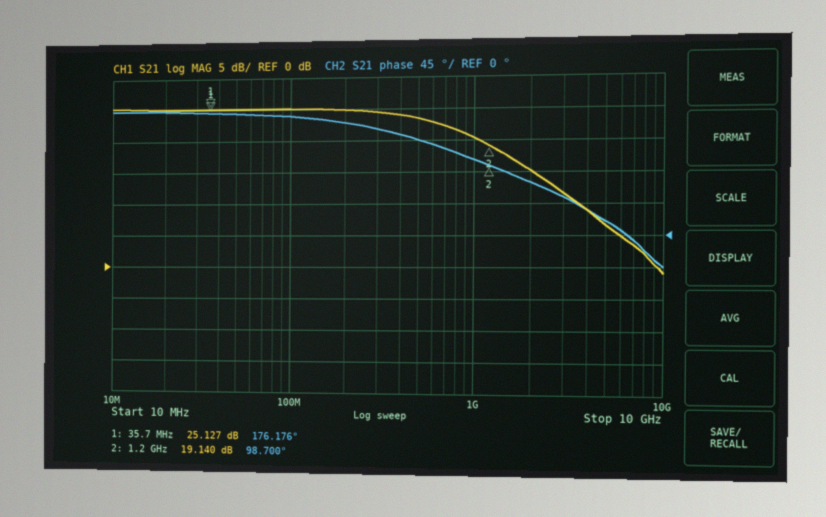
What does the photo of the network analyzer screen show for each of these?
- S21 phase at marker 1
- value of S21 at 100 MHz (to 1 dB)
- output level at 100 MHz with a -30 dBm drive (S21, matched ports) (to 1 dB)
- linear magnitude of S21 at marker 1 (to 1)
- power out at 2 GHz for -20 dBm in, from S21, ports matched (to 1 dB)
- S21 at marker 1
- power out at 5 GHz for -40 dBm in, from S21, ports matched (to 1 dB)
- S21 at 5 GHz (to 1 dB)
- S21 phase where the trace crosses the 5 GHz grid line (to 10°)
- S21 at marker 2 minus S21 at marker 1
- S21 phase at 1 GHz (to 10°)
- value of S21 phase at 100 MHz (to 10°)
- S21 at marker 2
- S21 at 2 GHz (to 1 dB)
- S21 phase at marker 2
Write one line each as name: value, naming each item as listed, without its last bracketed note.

S21 phase at marker 1: 176.176°
value of S21 at 100 MHz: 25 dB
output level at 100 MHz with a -30 dBm drive (S21, matched ports): -5 dBm
linear magnitude of S21 at marker 1: 18
power out at 2 GHz for -20 dBm in, from S21, ports matched: -5 dBm
S21 at marker 1: 25.127 dB
power out at 5 GHz for -40 dBm in, from S21, ports matched: -33 dBm
S21 at 5 GHz: 7 dB
S21 phase where the trace crosses the 5 GHz grid line: 20°
S21 at marker 2 minus S21 at marker 1: -5.987 dB
S21 phase at 1 GHz: 110°
value of S21 phase at 100 MHz: 170°
S21 at marker 2: 19.140 dB
S21 at 2 GHz: 15 dB
S21 phase at marker 2: 98.700°
